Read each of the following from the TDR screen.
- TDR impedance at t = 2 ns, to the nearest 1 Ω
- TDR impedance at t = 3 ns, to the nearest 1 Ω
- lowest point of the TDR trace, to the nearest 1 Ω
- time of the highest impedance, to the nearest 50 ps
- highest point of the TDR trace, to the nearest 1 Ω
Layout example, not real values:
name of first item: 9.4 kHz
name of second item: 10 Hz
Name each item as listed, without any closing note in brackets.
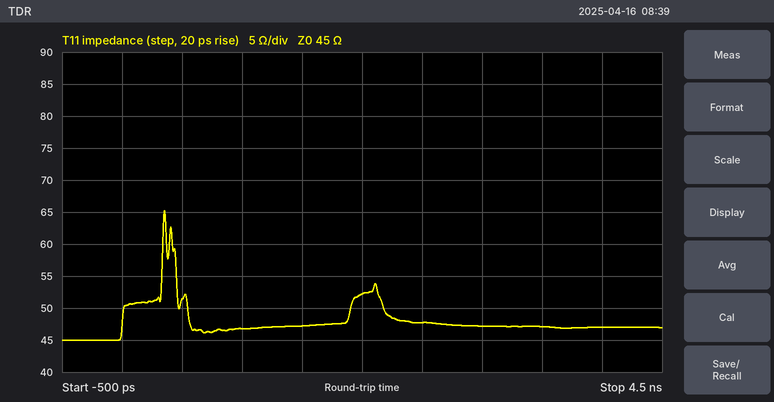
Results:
TDR impedance at t = 2 ns, to the nearest 1 Ω: 52 Ω
TDR impedance at t = 3 ns, to the nearest 1 Ω: 47 Ω
lowest point of the TDR trace, to the nearest 1 Ω: 45 Ω
time of the highest impedance, to the nearest 50 ps: 350 ps
highest point of the TDR trace, to the nearest 1 Ω: 65 Ω
